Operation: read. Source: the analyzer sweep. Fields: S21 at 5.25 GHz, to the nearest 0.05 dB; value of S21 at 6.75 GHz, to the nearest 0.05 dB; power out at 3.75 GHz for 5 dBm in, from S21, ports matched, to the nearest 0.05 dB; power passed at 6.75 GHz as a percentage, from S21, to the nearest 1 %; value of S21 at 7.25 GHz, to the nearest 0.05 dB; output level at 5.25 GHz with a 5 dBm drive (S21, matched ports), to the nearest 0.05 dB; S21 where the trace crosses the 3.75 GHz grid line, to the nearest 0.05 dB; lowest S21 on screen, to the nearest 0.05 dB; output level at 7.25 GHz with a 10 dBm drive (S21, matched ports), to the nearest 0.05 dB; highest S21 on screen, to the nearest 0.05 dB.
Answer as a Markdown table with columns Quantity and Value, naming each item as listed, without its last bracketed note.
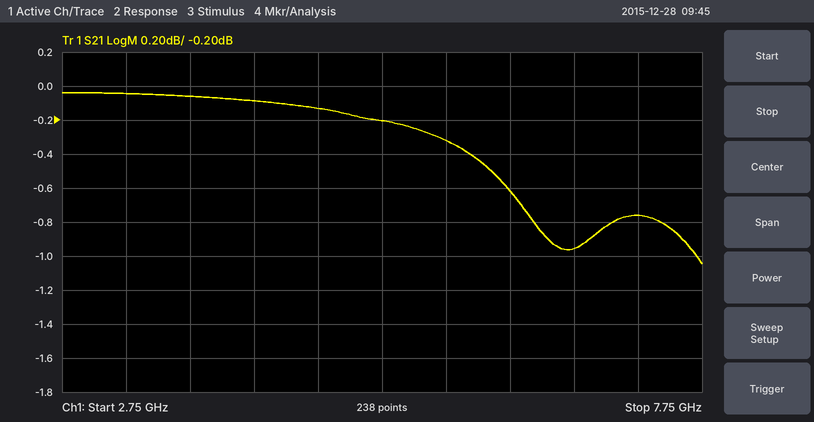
| Quantity | Value |
|---|---|
| S21 at 5.25 GHz, to the nearest 0.05 dB | -0.20 dB |
| value of S21 at 6.75 GHz, to the nearest 0.05 dB | -0.95 dB |
| power out at 3.75 GHz for 5 dBm in, from S21, ports matched, to the nearest 0.05 dB | 4.95 dBm |
| power passed at 6.75 GHz as a percentage, from S21, to the nearest 1 % | 80 % |
| value of S21 at 7.25 GHz, to the nearest 0.05 dB | -0.75 dB |
| output level at 5.25 GHz with a 5 dBm drive (S21, matched ports), to the nearest 0.05 dB | 4.80 dBm |
| S21 where the trace crosses the 3.75 GHz grid line, to the nearest 0.05 dB | -0.05 dB |
| lowest S21 on screen, to the nearest 0.05 dB | -1.05 dB |
| output level at 7.25 GHz with a 10 dBm drive (S21, matched ports), to the nearest 0.05 dB | 9.25 dBm |
| highest S21 on screen, to the nearest 0.05 dB | -0.05 dB |
